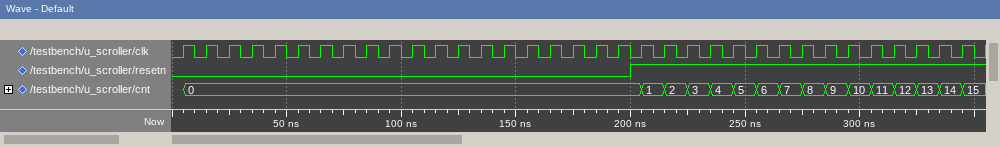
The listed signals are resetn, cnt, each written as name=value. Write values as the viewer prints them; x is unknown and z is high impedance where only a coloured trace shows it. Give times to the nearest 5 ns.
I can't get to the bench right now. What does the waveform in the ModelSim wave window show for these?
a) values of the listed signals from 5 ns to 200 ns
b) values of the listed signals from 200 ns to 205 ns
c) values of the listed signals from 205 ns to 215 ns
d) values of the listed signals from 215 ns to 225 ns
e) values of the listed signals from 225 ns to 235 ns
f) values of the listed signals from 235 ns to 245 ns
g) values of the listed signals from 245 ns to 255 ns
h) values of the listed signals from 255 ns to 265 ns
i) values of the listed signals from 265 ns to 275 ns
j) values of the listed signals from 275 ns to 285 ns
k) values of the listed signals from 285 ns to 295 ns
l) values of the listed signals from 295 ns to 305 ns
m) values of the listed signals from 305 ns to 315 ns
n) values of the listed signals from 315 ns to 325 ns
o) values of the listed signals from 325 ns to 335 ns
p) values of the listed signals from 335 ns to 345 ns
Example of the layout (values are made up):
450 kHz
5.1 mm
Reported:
resetn=0, cnt=0
resetn=1, cnt=0
resetn=1, cnt=1
resetn=1, cnt=2
resetn=1, cnt=3
resetn=1, cnt=4
resetn=1, cnt=5
resetn=1, cnt=6
resetn=1, cnt=7
resetn=1, cnt=8
resetn=1, cnt=9
resetn=1, cnt=10
resetn=1, cnt=11
resetn=1, cnt=12
resetn=1, cnt=13
resetn=1, cnt=14
